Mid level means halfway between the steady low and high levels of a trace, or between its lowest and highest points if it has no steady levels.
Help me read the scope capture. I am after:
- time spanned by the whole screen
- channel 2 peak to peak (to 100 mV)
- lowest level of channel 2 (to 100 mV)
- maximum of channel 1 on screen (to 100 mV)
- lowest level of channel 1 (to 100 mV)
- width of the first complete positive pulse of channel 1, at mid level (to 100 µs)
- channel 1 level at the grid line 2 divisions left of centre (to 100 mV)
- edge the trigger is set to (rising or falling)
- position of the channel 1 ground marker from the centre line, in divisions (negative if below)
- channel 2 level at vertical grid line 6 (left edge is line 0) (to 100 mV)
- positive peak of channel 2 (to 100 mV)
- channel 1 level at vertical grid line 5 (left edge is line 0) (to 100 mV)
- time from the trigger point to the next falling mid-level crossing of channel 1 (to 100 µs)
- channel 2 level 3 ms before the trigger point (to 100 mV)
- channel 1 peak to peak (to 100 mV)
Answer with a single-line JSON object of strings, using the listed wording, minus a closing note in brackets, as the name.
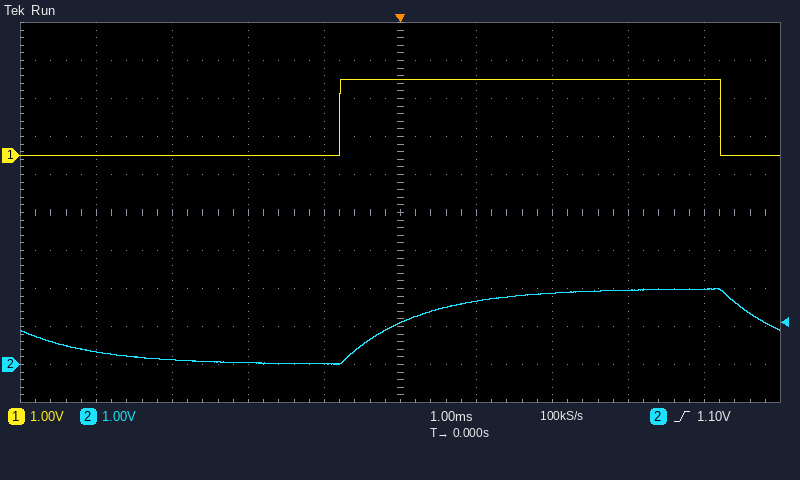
{"time spanned by the whole screen": "10 ms", "channel 2 peak to peak": "2.0 V", "lowest level of channel 2": "0.0 V", "maximum of channel 1 on screen": "2.0 V", "lowest level of channel 1": "0.0 V", "width of the first complete positive pulse of channel 1, at mid level": "5.0 ms", "channel 1 level at the grid line 2 divisions left of centre": "0.0 V", "edge the trigger is set to": "rising", "position of the channel 1 ground marker from the centre line, in divisions": "+1.5 div", "channel 2 level at vertical grid line 6 (left edge is line 0)": "1.7 V", "positive peak of channel 2": "2.0 V", "channel 1 level at vertical grid line 5 (left edge is line 0)": "2.0 V", "time from the trigger point to the next falling mid-level crossing of channel 1": "4.2 ms", "channel 2 level 3 ms before the trigger point": "100 mV", "channel 1 peak to peak": "2.0 V"}
